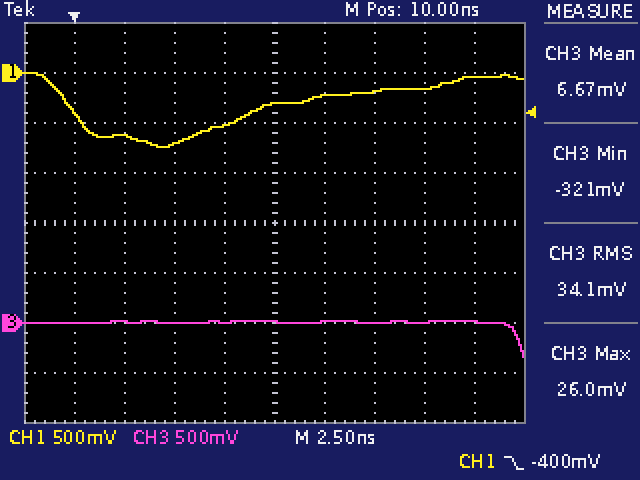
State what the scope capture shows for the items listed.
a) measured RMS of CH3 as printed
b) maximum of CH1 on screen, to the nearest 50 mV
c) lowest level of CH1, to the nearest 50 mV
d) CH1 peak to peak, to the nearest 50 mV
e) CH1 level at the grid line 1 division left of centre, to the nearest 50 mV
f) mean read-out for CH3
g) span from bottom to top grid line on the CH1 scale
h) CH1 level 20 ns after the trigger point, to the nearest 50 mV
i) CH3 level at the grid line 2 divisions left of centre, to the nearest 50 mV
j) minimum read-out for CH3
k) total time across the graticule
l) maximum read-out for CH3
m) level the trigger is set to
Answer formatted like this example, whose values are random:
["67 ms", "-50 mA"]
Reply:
["34.1 mV", "0 mV", "-750 mV", "750 mV", "-550 mV", "6.67 mV", "4 V", "-50 mV", "0 mV", "-321 mV", "25 ns", "26.0 mV", "-400 mV"]
